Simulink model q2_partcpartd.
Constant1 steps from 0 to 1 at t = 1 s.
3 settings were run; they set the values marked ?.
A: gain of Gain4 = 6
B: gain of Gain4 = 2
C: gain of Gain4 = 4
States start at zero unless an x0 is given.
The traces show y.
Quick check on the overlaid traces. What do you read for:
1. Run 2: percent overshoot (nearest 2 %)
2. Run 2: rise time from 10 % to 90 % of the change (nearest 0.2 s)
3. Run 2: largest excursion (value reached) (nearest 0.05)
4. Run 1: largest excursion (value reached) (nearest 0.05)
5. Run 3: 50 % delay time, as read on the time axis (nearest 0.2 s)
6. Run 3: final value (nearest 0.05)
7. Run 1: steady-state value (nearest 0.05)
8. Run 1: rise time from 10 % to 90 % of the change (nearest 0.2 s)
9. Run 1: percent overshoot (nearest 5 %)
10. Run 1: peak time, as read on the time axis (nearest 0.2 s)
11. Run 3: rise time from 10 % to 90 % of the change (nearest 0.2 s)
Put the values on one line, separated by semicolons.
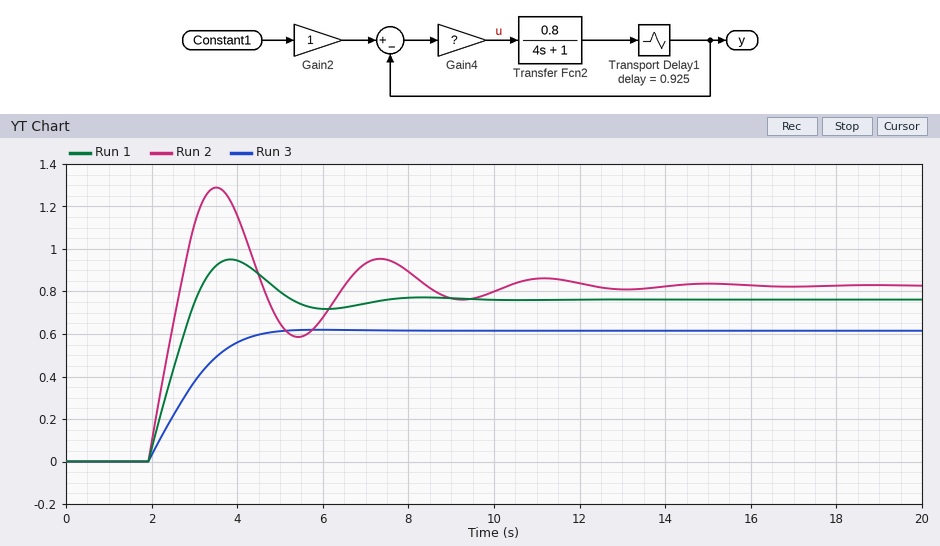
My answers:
56 %; 0.6 s; 1.30; 0.95; 2.8 s; 0.60; 0.75; 0.8 s; 25 %; 3.8 s; 1.8 s
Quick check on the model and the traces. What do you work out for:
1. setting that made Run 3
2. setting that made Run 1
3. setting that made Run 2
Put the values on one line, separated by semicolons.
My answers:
B; C; A
